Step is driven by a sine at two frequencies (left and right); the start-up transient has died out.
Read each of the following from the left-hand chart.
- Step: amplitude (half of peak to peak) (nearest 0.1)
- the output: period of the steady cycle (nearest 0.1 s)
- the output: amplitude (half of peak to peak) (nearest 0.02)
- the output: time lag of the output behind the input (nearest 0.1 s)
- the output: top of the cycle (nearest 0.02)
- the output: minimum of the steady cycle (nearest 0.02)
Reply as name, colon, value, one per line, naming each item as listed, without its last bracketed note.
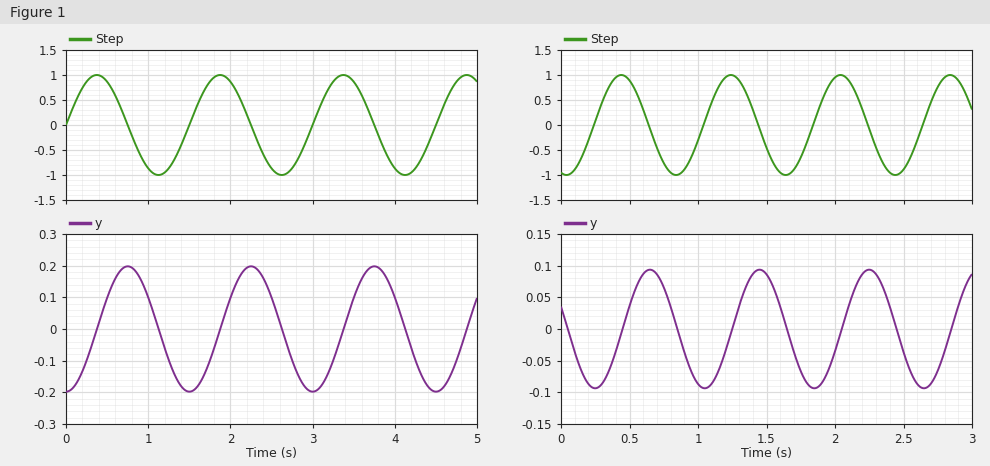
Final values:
Step: amplitude (half of peak to peak): 1.0
the output: period of the steady cycle: 1.5 s
the output: amplitude (half of peak to peak): 0.20
the output: time lag of the output behind the input: 0.4 s
the output: top of the cycle: 0.20
the output: minimum of the steady cycle: -0.20
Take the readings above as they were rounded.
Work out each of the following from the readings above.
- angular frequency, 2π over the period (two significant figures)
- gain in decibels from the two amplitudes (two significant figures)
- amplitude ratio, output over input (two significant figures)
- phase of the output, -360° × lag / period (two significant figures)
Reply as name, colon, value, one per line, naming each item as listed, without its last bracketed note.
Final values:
angular frequency, 2π over the period: 4.2 rad/s
gain in decibels from the two amplitudes: -14 dB
amplitude ratio, output over input: 0.20
phase of the output, -360° × lag / period: -96°
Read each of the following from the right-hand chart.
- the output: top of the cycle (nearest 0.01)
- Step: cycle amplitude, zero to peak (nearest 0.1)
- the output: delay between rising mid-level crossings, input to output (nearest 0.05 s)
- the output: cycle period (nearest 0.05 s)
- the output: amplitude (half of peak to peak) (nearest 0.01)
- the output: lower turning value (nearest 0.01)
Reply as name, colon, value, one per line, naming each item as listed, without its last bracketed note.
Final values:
the output: top of the cycle: 0.09
Step: cycle amplitude, zero to peak: 1.0
the output: delay between rising mid-level crossings, input to output: 0.20 s
the output: cycle period: 0.80 s
the output: amplitude (half of peak to peak): 0.09
the output: lower turning value: -0.09
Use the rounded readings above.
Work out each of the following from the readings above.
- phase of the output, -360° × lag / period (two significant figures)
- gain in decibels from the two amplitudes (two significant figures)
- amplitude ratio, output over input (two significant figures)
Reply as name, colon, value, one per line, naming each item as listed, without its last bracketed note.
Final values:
phase of the output, -360° × lag / period: -90°
gain in decibels from the two amplitudes: -21 dB
amplitude ratio, output over input: 0.090
